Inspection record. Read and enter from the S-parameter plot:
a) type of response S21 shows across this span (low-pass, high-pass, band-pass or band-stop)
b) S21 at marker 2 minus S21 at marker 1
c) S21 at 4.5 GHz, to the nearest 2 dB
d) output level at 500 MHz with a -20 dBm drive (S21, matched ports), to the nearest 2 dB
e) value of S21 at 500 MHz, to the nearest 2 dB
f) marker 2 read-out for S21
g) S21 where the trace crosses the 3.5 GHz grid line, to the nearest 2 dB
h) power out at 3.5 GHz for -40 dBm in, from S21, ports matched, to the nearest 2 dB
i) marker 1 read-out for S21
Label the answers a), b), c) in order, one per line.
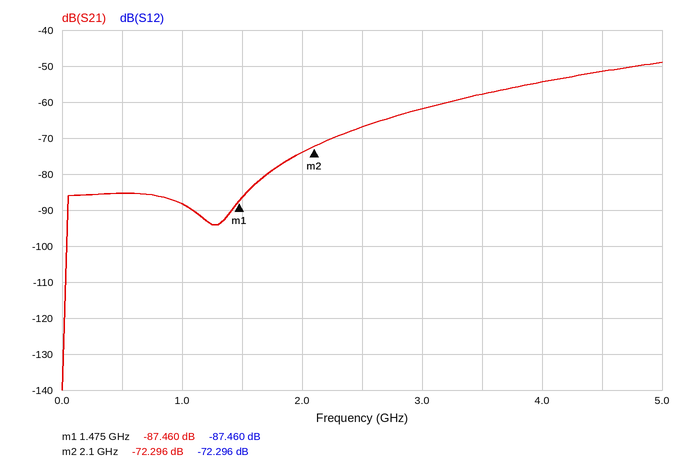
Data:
a) high-pass
b) 15.164 dB
c) -52 dB
d) -106 dBm
e) -86 dB
f) -72.296 dB
g) -58 dB
h) -98 dBm
i) -87.460 dB
